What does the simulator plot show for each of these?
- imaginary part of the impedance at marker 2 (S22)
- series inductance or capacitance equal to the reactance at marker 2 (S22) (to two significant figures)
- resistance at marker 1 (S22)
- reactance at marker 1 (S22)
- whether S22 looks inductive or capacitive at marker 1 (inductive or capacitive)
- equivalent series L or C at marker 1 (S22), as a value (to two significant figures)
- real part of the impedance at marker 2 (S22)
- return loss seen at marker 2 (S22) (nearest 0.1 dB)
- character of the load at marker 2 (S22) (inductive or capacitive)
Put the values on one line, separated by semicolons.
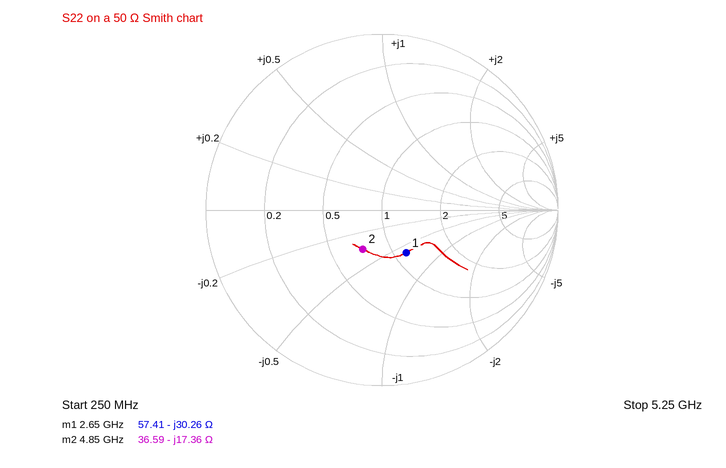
-17.36 Ω; 1.9 pF; 57.41 Ω; -30.26 Ω; capacitive; 2.0 pF; 36.59 Ω; 12.1 dB; capacitive
